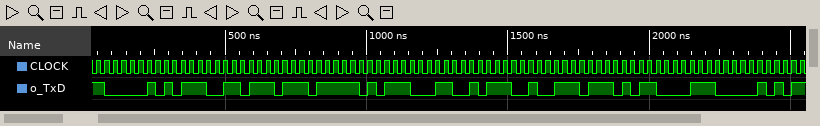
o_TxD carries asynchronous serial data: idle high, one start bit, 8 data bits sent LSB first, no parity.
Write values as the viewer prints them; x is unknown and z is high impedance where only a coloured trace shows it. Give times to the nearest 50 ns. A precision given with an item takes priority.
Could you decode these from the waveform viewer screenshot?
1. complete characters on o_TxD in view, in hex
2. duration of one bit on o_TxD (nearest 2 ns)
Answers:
50, 76, 5F, 4C, 72, 0D, 50
30 ns
